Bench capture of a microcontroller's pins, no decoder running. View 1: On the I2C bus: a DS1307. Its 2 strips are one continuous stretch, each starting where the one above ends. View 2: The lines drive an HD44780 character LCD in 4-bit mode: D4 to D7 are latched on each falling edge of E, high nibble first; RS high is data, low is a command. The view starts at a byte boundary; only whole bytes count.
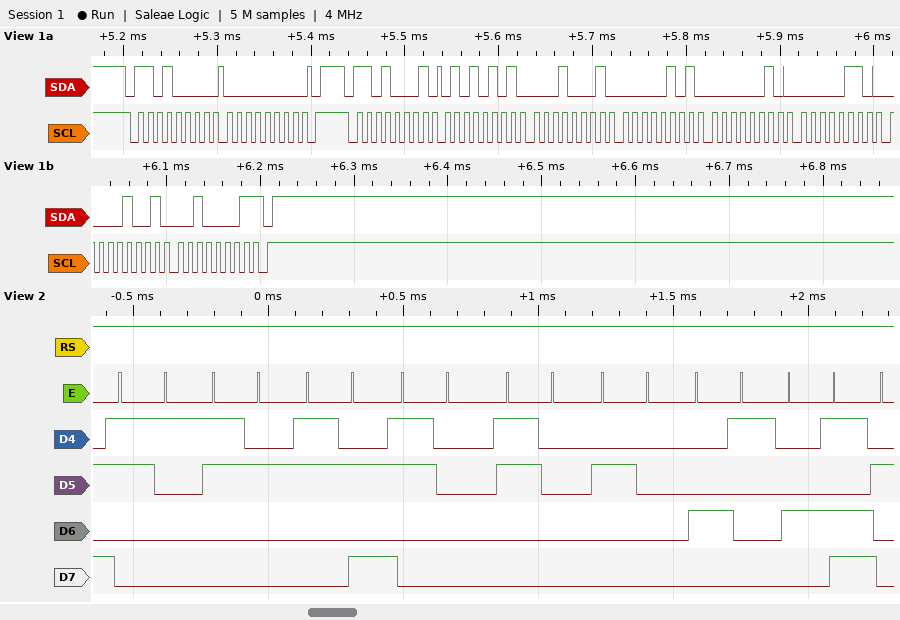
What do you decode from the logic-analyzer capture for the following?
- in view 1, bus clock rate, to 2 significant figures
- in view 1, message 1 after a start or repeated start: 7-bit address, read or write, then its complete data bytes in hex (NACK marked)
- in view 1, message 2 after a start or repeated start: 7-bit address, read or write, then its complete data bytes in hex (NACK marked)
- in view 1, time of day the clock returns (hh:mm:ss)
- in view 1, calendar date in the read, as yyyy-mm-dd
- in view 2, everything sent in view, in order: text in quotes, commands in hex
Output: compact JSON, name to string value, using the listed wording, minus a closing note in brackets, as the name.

{"in view 1, bus clock rate, to 2 significant figures": "100 kHz", "in view 1, message 1 after a start or repeated start: 7-bit address, read or write, then its complete data bytes in hex": "0x68 write: 00", "in view 1, message 2 after a start or repeated start: 7-bit address, read or write, then its complete data bytes in hex": "0x68 read: 55 11 05 02 06 09 21 NACK", "in view 1, time of day the clock returns": "05:11:55", "in view 1, calendar date in the read, as yyyy-mm-dd": "2021-09-06", "in view 2, everything sent in view, in order: text in quotes, commands in hex": "\"12:00 AM\""}
